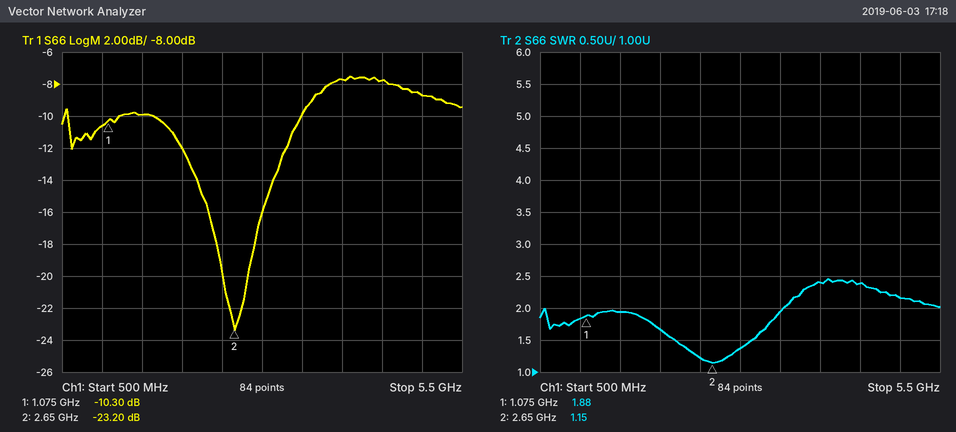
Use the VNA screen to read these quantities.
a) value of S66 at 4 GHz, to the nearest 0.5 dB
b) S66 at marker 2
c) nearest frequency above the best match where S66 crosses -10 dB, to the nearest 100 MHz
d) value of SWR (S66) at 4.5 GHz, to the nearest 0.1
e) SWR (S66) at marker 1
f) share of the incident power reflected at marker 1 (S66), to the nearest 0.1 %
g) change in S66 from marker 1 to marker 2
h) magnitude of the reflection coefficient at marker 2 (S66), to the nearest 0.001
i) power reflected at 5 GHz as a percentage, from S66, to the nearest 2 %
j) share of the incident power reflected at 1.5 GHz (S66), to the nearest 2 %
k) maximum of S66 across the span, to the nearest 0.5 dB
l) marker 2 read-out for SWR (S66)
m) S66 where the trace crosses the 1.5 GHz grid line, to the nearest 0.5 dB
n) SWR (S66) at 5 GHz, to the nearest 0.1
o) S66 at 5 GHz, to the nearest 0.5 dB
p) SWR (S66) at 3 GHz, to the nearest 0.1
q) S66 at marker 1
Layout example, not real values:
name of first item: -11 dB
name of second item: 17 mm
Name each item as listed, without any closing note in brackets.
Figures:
value of S66 at 4 GHz, to the nearest 0.5 dB: -7.5 dB
S66 at marker 2: -23.20 dB
nearest frequency above the best match where S66 crosses -10 dB, to the nearest 100 MHz: 3.5 GHz
value of SWR (S66) at 4.5 GHz, to the nearest 0.1: 2.4
SWR (S66) at marker 1: 1.88
share of the incident power reflected at marker 1 (S66), to the nearest 0.1 %: 9.3 %
change in S66 from marker 1 to marker 2: -12.90 dB
magnitude of the reflection coefficient at marker 2 (S66), to the nearest 0.001: 0.069
power reflected at 5 GHz as a percentage, from S66, to the nearest 2 %: 14 %
share of the incident power reflected at 1.5 GHz (S66), to the nearest 2 %: 10 %
maximum of S66 across the span, to the nearest 0.5 dB: -7.5 dB
marker 2 read-out for SWR: 1.15
S66 where the trace crosses the 1.5 GHz grid line, to the nearest 0.5 dB: -10.0 dB
SWR (S66) at 5 GHz, to the nearest 0.1: 2.2
S66 at 5 GHz, to the nearest 0.5 dB: -8.5 dB
SWR (S66) at 3 GHz, to the nearest 0.1: 1.4
S66 at marker 1: -10.30 dB
